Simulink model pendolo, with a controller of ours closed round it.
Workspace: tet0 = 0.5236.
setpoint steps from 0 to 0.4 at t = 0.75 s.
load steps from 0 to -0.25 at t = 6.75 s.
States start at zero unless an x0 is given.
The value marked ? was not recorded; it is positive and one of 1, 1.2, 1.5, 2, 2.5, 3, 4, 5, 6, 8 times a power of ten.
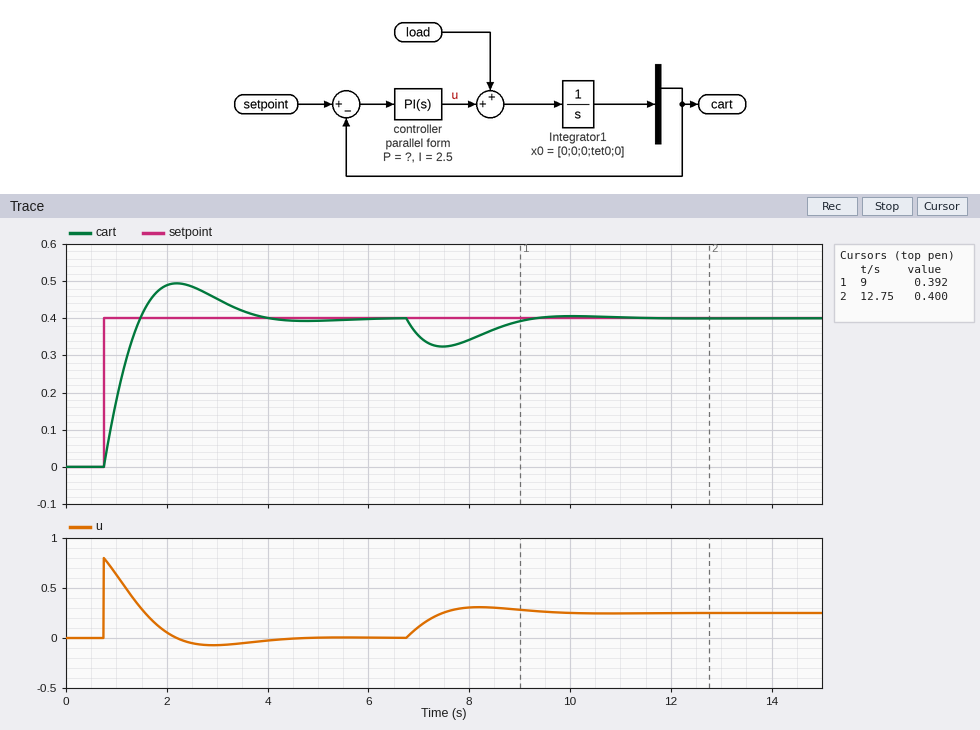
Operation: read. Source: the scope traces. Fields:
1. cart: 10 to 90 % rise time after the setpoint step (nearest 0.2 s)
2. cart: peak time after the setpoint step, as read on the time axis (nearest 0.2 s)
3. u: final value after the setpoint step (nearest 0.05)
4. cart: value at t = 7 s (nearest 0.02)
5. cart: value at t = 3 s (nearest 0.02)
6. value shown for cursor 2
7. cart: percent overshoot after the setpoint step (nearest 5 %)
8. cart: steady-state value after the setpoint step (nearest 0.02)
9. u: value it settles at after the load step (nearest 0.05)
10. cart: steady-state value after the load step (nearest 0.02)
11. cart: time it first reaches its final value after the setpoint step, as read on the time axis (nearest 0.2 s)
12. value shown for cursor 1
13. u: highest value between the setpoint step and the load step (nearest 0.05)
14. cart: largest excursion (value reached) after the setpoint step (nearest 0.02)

0.6 s
2.2 s
0.00
0.36
0.46
0.400
25 %
0.40
0.25
0.40
1.4 s
0.392
0.80
0.50
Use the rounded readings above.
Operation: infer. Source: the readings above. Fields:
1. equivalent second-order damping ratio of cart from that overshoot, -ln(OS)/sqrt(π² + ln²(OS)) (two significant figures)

0.40
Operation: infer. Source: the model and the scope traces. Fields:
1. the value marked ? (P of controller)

2
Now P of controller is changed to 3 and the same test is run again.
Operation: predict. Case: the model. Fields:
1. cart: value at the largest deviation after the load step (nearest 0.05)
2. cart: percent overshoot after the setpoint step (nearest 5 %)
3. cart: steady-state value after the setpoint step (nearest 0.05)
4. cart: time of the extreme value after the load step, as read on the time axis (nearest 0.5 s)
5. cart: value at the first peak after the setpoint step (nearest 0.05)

0.35
15 %
0.40
7.5 s
0.45
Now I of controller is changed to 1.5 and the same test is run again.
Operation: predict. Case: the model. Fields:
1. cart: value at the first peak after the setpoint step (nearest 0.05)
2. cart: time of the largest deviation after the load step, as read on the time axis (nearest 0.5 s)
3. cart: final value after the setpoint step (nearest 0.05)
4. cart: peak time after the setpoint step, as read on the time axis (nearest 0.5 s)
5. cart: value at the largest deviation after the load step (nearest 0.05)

0.45
7.5 s
0.40
2.5 s
0.30
